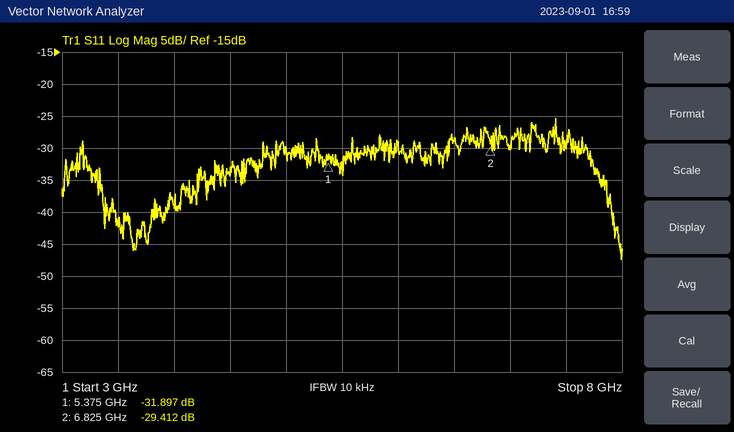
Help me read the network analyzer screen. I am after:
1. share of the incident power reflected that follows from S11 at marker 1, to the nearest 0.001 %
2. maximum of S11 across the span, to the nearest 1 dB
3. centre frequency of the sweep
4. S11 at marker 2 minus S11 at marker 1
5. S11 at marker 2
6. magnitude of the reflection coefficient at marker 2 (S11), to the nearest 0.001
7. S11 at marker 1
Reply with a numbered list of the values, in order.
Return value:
1. 0.065 %
2. -25 dB
3. 5.5 GHz
4. 2.485 dB
5. -29.412 dB
6. 0.034
7. -31.897 dB
